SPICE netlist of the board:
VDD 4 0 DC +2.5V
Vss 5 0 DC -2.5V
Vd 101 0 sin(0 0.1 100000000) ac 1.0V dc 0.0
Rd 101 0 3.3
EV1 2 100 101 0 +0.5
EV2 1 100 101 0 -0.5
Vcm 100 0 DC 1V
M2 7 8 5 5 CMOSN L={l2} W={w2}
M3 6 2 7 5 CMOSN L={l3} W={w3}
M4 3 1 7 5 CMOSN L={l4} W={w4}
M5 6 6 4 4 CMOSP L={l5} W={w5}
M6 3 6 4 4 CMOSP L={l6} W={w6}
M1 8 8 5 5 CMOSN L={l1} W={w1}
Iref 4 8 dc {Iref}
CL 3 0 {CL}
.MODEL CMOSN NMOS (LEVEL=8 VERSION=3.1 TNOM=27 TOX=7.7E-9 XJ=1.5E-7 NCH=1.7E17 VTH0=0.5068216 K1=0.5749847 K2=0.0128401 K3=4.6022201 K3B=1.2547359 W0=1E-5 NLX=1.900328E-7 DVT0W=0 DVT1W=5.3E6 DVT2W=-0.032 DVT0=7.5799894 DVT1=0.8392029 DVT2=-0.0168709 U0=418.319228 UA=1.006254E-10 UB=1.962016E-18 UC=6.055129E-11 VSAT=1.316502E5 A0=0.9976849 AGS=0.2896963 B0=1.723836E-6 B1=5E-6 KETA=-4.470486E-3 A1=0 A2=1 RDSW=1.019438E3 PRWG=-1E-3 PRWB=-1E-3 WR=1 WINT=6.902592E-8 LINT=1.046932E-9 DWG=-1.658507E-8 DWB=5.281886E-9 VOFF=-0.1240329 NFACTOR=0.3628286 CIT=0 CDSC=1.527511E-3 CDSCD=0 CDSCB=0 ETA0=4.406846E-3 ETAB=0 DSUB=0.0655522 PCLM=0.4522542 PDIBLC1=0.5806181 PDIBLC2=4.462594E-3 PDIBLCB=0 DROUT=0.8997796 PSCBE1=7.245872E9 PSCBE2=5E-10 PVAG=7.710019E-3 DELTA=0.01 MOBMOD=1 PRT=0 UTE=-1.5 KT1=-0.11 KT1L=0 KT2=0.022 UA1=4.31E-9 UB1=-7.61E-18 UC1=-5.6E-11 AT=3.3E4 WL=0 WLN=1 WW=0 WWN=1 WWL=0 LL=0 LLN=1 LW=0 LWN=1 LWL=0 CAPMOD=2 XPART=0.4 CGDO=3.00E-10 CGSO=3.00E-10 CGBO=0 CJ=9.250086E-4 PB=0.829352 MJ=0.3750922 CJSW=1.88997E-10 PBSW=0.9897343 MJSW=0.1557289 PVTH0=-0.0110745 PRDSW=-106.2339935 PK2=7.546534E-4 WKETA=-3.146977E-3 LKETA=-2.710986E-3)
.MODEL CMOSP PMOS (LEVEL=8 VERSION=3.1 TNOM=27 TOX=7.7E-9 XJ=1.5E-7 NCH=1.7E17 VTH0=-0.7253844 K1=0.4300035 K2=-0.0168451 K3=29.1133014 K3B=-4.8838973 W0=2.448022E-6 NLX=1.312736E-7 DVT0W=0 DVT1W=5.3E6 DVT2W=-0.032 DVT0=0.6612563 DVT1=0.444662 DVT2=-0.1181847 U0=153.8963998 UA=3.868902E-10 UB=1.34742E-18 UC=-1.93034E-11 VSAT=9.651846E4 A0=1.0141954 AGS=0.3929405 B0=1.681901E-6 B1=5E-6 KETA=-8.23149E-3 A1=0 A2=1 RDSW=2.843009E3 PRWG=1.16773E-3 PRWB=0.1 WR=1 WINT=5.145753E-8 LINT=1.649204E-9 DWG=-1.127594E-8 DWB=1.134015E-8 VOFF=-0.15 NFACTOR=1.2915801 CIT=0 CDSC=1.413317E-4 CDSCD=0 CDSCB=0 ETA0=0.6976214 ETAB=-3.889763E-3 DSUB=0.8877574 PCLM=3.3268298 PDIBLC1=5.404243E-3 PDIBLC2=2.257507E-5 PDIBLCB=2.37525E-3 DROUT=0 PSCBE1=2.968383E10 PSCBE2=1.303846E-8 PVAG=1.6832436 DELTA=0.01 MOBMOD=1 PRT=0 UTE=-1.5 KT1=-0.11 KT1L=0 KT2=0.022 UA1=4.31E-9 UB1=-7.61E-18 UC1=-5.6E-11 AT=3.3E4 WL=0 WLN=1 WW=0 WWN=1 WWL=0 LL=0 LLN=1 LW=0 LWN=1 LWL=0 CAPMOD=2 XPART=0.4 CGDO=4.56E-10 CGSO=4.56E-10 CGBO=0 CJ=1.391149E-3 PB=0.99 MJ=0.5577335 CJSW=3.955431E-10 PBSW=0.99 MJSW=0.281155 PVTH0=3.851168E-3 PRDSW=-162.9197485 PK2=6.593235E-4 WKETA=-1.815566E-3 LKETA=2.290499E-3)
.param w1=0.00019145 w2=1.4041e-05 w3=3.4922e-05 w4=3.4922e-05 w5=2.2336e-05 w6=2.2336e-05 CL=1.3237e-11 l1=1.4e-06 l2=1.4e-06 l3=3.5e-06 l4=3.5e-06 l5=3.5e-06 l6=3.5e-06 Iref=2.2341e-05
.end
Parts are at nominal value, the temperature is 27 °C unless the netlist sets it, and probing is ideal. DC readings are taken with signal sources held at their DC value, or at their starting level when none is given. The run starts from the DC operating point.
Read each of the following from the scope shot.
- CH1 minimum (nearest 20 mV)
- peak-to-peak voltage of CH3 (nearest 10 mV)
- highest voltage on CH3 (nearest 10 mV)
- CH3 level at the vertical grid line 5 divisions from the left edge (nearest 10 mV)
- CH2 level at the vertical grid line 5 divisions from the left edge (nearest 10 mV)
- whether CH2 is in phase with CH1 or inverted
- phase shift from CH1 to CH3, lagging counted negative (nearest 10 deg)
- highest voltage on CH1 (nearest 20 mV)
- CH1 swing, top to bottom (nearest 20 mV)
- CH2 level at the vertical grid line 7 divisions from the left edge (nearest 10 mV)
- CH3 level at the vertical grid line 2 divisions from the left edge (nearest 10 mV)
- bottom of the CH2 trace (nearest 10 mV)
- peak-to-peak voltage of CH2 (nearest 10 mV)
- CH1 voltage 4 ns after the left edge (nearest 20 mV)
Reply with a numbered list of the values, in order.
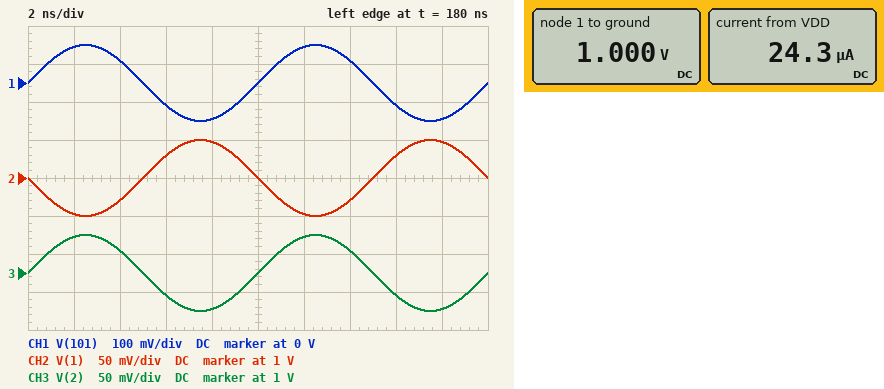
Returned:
1. -100 mV
2. 100 mV
3. 1.05 V
4. 1.00 V
5. 1.00 V
6. inverted
7. 0 deg
8. 100 mV
9. 200 mV
10. 970 mV
11. 1.03 V
12. 950 mV
13. 100 mV
14. 60 mV
